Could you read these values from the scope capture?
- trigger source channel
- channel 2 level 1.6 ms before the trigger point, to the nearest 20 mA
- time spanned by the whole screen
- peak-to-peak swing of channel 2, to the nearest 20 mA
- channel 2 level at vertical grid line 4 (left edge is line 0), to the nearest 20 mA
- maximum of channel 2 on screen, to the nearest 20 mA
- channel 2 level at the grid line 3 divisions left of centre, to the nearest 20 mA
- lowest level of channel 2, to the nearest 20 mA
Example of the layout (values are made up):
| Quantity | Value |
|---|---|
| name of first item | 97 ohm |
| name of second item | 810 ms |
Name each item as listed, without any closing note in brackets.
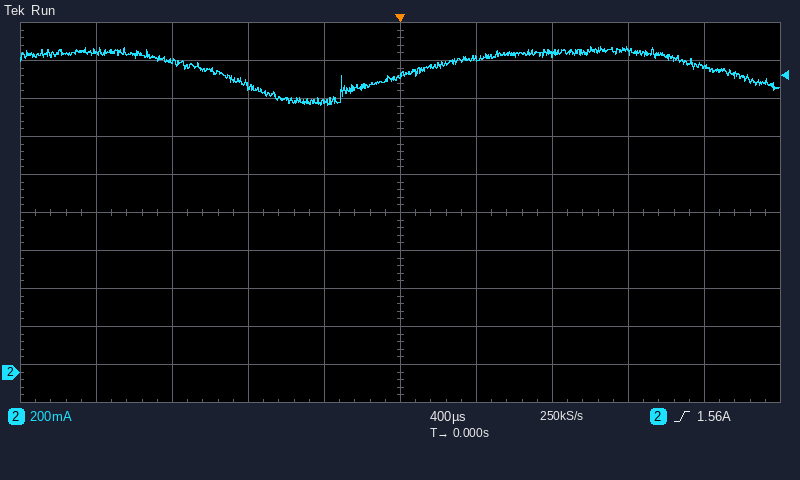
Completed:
| Quantity | Value |
|---|---|
| trigger source channel | channel 2 |
| channel 2 level 1.6 ms before the trigger point, to the nearest 20 mA | 1.68 A |
| time spanned by the whole screen | 4 ms |
| peak-to-peak swing of channel 2, to the nearest 20 mA | 320 mA |
| channel 2 level at vertical grid line 4 (left edge is line 0), to the nearest 20 mA | 1.42 A |
| maximum of channel 2 on screen, to the nearest 20 mA | 1.72 A |
| channel 2 level at the grid line 3 divisions left of centre, to the nearest 20 mA | 1.64 A |
| lowest level of channel 2, to the nearest 20 mA | 1.40 A |
